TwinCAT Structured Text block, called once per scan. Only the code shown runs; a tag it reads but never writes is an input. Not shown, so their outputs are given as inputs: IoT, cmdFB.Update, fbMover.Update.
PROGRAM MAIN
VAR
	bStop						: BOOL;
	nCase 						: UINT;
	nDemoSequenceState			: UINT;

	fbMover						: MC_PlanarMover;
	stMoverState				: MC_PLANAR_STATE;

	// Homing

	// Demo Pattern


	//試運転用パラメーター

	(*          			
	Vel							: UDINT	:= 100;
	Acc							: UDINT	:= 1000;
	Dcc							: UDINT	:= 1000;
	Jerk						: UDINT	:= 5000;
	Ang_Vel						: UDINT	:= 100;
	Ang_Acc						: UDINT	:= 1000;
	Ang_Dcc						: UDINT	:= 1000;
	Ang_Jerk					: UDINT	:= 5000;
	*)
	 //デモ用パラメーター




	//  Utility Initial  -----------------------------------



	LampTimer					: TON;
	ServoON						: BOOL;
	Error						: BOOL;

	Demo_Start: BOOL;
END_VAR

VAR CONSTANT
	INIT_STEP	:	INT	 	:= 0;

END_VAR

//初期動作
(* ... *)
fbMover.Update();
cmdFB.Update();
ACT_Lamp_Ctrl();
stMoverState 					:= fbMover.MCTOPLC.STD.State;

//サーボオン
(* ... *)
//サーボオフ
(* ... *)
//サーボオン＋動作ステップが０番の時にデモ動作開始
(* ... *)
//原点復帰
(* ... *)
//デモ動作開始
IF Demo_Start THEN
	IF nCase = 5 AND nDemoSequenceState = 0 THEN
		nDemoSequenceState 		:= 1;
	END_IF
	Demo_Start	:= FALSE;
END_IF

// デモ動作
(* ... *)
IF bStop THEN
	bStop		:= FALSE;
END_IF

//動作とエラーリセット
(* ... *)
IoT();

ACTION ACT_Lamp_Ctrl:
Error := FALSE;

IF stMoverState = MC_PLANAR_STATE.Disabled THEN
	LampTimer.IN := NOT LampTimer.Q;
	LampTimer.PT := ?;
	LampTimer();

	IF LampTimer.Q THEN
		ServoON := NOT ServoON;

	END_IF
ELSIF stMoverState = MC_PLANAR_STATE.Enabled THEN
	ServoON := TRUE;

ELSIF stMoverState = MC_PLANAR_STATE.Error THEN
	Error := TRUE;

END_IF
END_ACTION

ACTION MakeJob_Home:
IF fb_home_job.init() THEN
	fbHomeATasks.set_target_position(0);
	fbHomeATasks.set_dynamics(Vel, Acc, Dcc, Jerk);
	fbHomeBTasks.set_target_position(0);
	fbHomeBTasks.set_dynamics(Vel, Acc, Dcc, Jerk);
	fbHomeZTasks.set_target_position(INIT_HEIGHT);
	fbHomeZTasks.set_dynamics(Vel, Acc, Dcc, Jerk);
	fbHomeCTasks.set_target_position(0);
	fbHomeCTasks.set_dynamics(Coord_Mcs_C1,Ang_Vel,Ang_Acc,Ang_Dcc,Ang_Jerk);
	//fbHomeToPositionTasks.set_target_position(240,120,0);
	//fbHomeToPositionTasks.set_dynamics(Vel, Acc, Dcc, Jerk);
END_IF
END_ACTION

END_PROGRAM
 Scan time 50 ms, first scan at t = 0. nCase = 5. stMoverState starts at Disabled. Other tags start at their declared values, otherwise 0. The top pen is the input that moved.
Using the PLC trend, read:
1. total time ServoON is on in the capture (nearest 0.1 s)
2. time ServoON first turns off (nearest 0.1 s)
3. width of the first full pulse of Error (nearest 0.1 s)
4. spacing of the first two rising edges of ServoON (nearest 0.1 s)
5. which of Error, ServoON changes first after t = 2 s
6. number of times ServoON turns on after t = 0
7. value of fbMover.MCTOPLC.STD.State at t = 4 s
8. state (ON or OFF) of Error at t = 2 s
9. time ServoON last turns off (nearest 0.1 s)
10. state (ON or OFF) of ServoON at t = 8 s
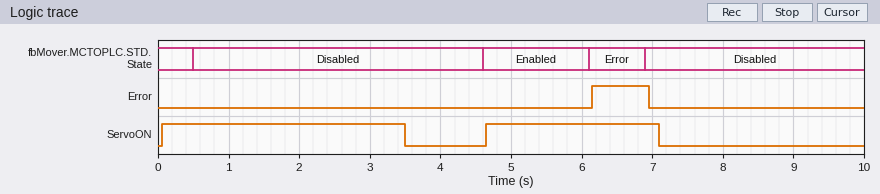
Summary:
5.9 s
3.5 s
0.8 s
4.6 s
ServoON
2
Disabled
OFF
7.1 s
OFF
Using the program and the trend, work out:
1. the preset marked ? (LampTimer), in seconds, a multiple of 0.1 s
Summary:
3.5 s
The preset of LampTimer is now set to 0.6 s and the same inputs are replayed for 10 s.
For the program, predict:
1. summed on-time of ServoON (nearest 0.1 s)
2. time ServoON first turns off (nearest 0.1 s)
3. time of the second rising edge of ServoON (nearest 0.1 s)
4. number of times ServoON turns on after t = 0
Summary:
6.2 s
0.6 s
1.3 s
6
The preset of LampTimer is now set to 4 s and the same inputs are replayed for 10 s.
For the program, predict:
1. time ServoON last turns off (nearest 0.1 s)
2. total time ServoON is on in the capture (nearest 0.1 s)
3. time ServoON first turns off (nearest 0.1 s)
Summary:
8.1 s
7.4 s
4.0 s
